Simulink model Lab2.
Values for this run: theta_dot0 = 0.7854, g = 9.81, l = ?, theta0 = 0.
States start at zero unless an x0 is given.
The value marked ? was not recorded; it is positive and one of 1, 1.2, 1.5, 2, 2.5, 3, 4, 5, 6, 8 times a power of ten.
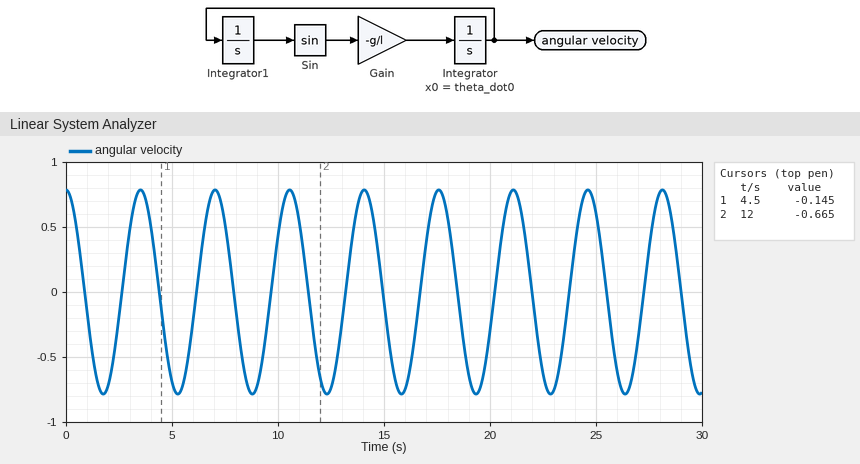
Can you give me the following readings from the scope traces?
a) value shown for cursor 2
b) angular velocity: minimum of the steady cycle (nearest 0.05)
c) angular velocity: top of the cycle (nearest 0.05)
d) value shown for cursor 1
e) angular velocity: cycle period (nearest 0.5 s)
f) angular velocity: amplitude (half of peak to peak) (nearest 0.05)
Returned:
-0.665
-0.80
0.80
-0.145
3.5 s
0.80
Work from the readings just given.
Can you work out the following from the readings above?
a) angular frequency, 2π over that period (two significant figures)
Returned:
1.8 rad/s
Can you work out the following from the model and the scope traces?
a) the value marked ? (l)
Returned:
3
